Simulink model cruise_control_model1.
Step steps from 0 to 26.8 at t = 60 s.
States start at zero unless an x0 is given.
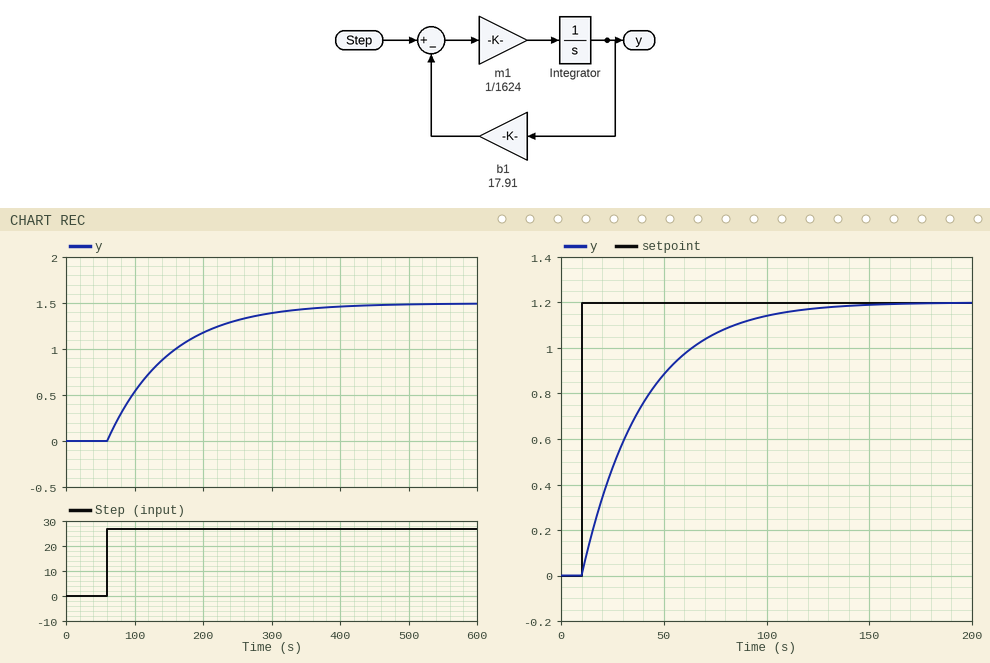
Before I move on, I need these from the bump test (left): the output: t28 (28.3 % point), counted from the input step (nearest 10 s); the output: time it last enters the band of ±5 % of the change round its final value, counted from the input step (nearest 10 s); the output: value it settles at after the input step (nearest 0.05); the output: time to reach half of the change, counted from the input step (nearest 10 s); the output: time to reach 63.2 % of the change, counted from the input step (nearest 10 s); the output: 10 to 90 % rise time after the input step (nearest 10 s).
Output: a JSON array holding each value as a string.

["30 s", "270 s", "1.50", "60 s", "90 s", "200 s"]
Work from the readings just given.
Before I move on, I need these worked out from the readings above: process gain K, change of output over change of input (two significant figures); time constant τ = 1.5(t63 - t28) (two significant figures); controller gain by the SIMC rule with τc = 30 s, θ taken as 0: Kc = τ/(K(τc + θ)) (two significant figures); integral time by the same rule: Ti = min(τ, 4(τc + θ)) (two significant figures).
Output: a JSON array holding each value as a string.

["0.056", "90 s", "54", "90 s"]
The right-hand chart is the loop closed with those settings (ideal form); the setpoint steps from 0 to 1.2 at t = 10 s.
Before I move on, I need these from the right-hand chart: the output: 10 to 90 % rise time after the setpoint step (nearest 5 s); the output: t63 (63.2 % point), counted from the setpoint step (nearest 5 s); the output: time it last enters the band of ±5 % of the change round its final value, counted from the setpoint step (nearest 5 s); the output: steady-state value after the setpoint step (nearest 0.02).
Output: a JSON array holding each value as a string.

["65 s", "30 s", "90 s", "1.20"]
